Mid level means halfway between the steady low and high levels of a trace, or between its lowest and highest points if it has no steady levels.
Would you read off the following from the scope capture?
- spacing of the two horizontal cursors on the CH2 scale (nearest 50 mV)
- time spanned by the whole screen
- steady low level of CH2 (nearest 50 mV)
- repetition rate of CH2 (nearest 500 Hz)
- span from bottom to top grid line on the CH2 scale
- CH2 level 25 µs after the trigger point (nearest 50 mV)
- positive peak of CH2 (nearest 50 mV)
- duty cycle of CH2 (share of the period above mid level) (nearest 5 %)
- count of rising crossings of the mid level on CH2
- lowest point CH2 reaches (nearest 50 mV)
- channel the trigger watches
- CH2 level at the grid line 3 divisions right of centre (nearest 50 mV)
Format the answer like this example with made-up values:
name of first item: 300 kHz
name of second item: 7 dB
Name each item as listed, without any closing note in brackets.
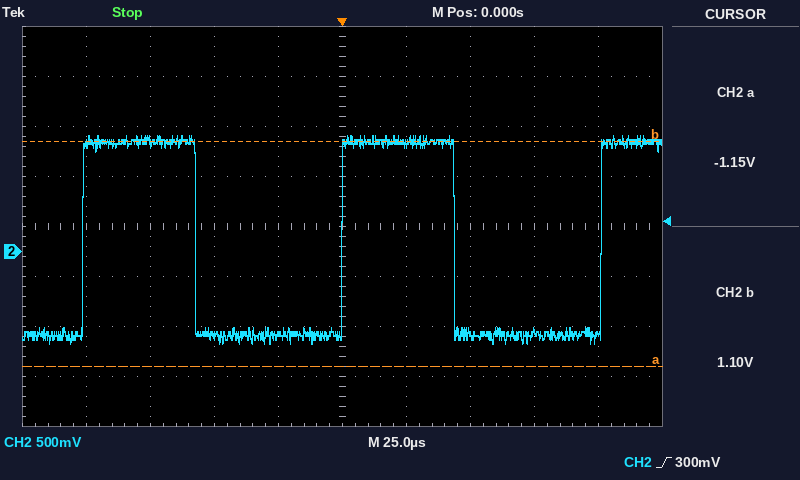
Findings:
spacing of the two horizontal cursors on the CH2 scale: 2.25 V
time spanned by the whole screen: 250 µs
steady low level of CH2: -850 mV
repetition rate of CH2: 10.0 kHz
span from bottom to top grid line on the CH2 scale: 4 V
CH2 level 25 µs after the trigger point: 1.10 V
positive peak of CH2: 1.15 V
duty cycle of CH2 (share of the period above mid level): 45 %
count of rising crossings of the mid level on CH2: 3
lowest point CH2 reaches: -900 mV
channel the trigger watches: CH2
CH2 level at the grid line 3 divisions right of centre: -800 mV
